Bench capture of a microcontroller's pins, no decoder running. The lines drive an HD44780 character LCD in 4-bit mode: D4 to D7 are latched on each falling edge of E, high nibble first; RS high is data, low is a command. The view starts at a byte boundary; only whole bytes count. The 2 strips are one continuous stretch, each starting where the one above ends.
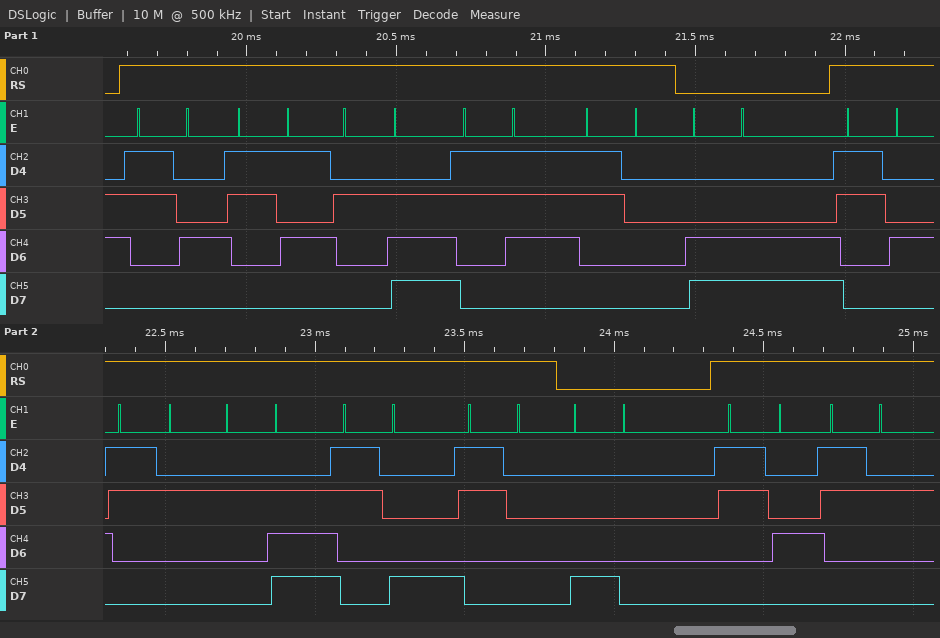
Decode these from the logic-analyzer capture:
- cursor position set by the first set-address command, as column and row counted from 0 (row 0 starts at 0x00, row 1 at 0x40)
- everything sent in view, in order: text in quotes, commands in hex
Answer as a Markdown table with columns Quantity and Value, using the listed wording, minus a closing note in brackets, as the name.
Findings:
| Quantity | Value |
|---|---|
| cursor position set by the first set-address command, as column and row counted from 0 | column 12, row 1 |
| everything sent in view, in order: text in quotes, commands in hex | "45.70" 0xCC "42.80" 0x80 "42" |
